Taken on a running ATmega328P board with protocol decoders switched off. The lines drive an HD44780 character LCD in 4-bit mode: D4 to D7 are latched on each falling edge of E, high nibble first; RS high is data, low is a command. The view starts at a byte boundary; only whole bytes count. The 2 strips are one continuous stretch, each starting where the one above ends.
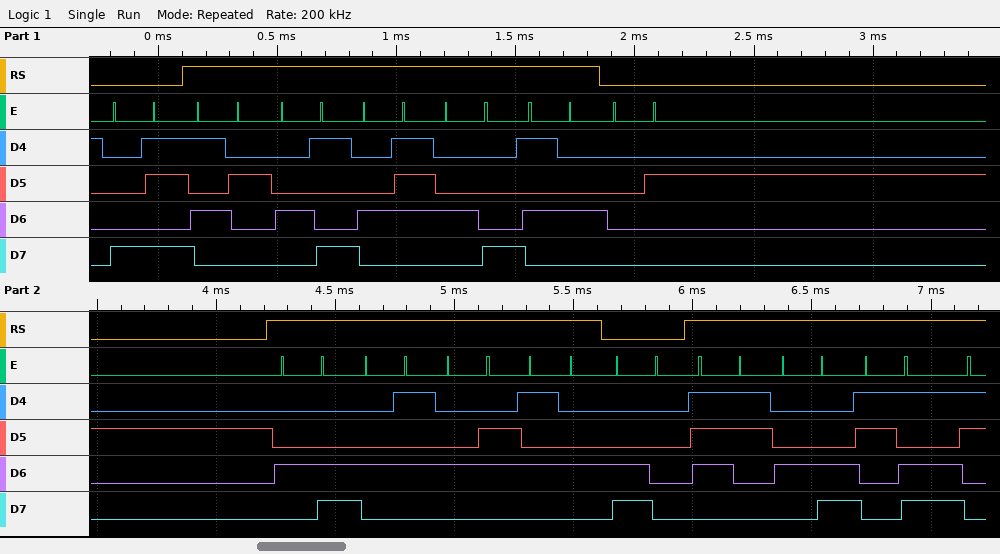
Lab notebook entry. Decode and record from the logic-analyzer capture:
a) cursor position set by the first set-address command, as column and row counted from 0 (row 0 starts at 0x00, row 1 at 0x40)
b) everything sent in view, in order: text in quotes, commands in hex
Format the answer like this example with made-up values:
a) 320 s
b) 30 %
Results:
a) column 11, row 0
b) 0x8B "RIGHT" 0x02 "LEFT" 0xC0 "sL="
